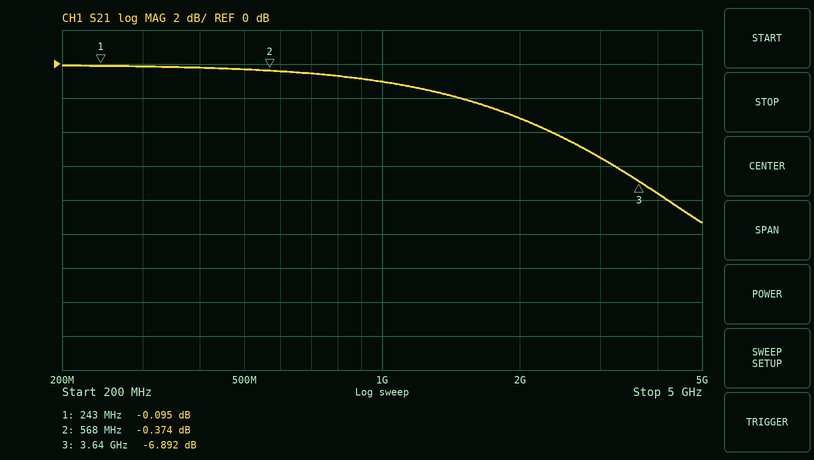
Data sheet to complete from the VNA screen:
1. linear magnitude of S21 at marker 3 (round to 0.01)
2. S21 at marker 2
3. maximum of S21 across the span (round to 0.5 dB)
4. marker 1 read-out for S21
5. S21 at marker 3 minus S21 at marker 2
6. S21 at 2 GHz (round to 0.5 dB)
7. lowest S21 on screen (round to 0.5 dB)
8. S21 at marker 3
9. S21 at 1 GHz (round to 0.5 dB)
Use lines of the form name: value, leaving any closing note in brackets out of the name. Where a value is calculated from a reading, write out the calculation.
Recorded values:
linear magnitude of S21 at marker 3: 10^(-6.892/20) ≈ 0.45
S21 at marker 2: -0.374 dB
maximum of S21 across the span: 0.0 dB
marker 1 read-out for S21: -0.095 dB
S21 at marker 3 minus S21 at marker 2: -6.892 − (-0.374) = -6.518 dB
S21 at 2 GHz: -3.0 dB
lowest S21 on screen: -9.5 dB
S21 at marker 3: -6.892 dB
S21 at 1 GHz: -1.0 dB
